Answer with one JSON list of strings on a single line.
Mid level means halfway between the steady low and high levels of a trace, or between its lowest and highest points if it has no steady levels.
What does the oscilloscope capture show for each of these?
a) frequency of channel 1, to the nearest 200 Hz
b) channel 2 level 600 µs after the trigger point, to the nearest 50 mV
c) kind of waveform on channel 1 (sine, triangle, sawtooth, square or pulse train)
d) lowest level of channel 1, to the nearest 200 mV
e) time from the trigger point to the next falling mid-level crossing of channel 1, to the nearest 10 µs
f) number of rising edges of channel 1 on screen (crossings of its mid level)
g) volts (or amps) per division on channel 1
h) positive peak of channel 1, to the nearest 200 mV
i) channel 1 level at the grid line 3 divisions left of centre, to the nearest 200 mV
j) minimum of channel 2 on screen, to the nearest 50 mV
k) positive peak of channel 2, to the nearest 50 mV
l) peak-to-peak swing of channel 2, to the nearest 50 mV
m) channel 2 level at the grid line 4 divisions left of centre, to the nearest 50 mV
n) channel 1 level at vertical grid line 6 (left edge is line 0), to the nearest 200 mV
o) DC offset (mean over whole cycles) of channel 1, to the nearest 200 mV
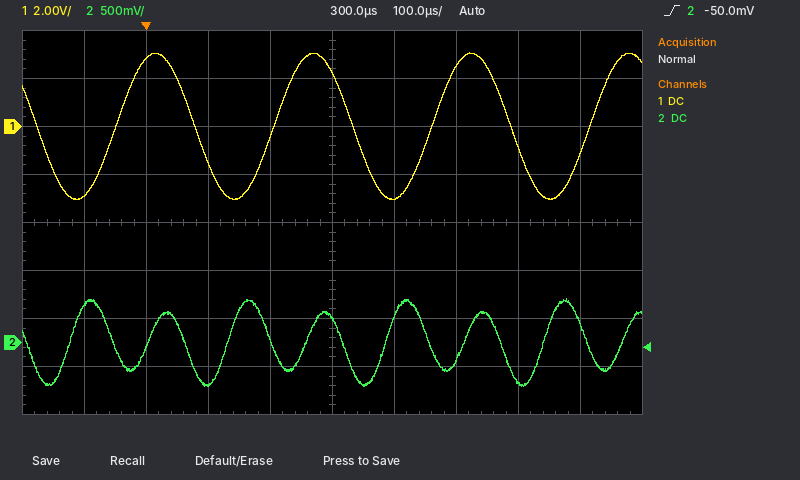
["4.0 kHz", "-400 mV", "sine", "-3.0 V", "80 µs", "4", "2 V", "3.0 V", "2.8 V", "-450 mV", "450 mV", "900 mV", "400 mV", "-3.0 V", "0.0 V"]
